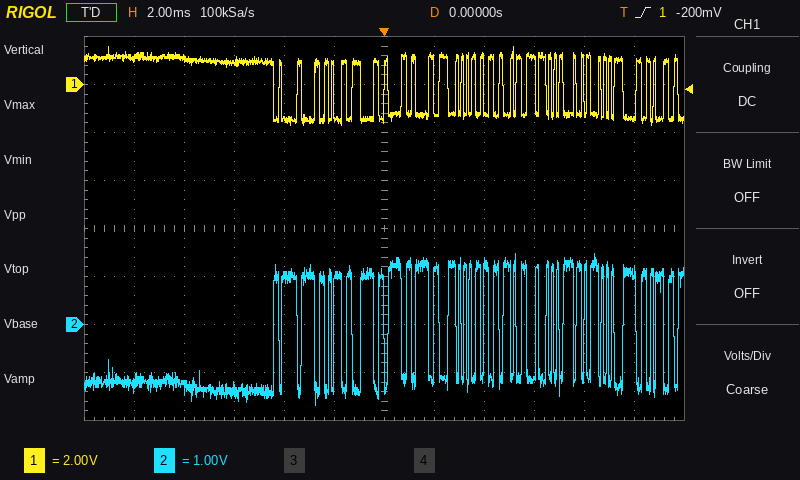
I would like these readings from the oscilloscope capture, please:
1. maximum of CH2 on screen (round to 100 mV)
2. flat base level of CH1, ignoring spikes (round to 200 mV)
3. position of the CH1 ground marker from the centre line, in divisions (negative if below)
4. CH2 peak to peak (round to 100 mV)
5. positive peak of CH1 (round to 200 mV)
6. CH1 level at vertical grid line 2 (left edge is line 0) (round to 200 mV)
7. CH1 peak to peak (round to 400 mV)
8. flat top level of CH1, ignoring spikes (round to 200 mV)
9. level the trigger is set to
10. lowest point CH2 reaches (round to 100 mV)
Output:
1.5 V
-1.4 V
+3.0 div
3.2 V
1.6 V
1.0 V
3.2 V
1.0 V
-200 mV
-1.7 V
